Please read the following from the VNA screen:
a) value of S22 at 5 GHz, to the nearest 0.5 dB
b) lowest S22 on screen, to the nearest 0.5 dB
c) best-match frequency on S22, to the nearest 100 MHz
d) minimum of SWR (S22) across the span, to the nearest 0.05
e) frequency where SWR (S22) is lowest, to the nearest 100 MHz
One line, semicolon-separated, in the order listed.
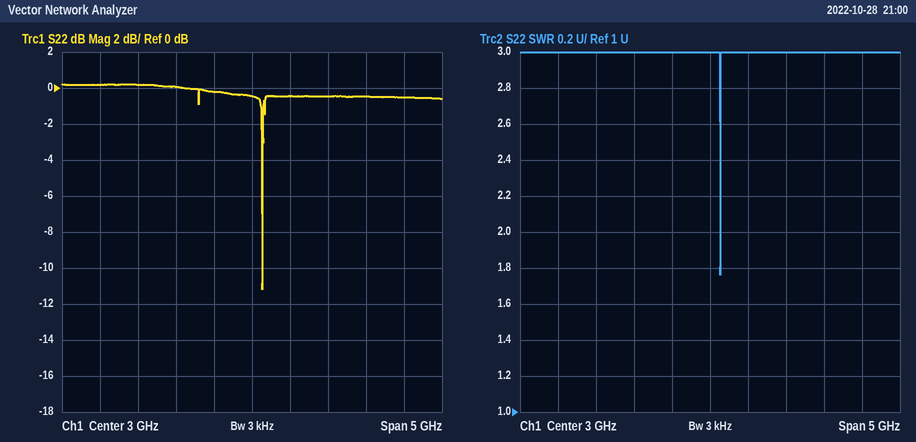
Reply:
-0.5 dB; -11.0 dB; 3.1 GHz; 1.75; 3.1 GHz
